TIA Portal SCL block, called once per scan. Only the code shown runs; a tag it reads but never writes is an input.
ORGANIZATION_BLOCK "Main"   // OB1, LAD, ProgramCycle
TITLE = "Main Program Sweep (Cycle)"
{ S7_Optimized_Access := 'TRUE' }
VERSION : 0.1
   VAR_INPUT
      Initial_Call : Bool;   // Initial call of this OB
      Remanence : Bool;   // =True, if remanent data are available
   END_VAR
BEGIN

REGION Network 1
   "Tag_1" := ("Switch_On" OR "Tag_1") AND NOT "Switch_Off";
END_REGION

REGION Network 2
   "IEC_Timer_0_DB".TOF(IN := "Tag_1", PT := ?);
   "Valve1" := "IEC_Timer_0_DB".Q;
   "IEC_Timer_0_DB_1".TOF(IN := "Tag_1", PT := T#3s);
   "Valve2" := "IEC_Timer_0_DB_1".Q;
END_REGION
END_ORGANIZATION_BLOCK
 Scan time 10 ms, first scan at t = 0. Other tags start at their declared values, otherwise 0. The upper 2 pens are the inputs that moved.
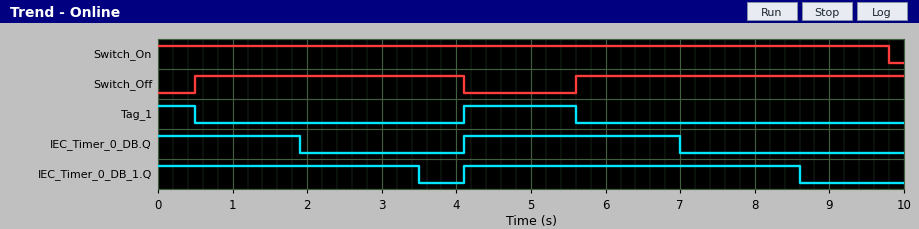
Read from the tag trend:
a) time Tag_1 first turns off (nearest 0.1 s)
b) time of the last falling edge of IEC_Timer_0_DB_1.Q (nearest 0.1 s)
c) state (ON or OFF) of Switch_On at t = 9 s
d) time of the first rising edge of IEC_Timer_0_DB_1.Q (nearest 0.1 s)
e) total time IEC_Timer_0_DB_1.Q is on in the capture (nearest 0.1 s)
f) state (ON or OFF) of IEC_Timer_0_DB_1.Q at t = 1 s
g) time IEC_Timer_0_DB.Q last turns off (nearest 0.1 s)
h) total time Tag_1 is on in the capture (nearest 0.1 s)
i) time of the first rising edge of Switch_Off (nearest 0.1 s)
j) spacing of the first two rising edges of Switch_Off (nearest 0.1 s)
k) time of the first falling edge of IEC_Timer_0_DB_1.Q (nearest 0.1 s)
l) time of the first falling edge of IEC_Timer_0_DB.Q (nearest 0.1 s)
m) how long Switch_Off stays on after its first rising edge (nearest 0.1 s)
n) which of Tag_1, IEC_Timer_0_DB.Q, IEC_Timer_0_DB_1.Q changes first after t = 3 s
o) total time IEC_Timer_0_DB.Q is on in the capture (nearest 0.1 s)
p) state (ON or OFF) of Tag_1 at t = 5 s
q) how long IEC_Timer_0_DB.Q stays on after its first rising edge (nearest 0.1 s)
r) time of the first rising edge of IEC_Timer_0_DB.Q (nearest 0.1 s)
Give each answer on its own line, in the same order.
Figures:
0.5 s
8.6 s
ON
4.1 s
8.0 s
ON
7.0 s
2.0 s
0.5 s
5.1 s
3.5 s
1.9 s
3.6 s
IEC_Timer_0_DB_1.Q
4.8 s
ON
2.9 s
4.1 s
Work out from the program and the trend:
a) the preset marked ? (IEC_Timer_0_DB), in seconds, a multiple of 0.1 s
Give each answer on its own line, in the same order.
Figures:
1.4 s
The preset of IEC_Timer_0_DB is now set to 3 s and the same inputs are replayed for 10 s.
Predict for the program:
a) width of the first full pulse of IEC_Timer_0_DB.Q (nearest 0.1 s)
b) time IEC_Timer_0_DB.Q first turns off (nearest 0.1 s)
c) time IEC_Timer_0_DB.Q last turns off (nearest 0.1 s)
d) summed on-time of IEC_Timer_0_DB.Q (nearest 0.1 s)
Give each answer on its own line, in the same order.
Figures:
4.5 s
3.5 s
8.6 s
8.0 s
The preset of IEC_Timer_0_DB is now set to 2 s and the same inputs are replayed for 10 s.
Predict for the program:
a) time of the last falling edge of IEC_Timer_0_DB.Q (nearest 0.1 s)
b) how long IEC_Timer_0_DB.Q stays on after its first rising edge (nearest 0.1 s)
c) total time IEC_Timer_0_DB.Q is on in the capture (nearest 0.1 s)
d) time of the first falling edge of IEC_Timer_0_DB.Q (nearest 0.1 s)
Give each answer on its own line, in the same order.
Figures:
7.6 s
3.5 s
6.0 s
2.5 s
